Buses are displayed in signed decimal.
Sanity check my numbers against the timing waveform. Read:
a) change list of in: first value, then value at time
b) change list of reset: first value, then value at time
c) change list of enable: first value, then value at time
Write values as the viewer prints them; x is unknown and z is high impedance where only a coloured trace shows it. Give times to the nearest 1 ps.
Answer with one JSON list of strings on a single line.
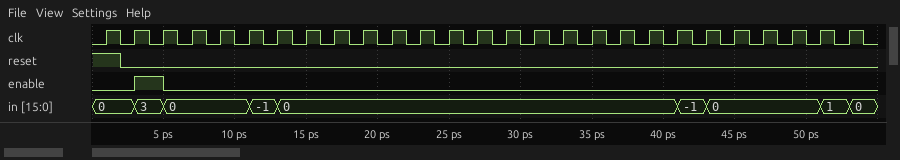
["0, 3 at 3 ps, 0 at 5 ps, -1 at 11 ps, 0 at 13 ps, -1 at 41 ps, 0 at 43 ps, 1 at 51 ps, 0 at 53 ps", "1, 0 at 2 ps", "0, 1 at 3 ps, 0 at 5 ps"]
